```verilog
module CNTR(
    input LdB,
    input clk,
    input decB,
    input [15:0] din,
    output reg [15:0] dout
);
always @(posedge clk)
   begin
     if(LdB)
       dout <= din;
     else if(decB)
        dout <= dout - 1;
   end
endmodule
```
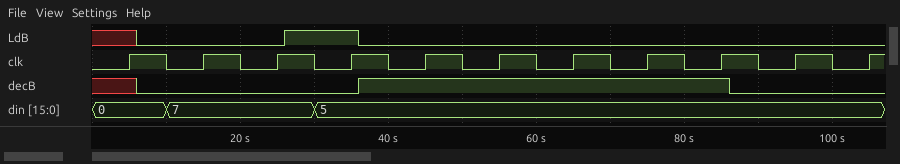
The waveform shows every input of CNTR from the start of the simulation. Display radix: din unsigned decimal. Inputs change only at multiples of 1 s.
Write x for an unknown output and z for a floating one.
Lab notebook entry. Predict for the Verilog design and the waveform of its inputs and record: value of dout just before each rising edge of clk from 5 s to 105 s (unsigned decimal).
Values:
x, x, x, x, 5, 4, 3, 2, 1, 0, 0
